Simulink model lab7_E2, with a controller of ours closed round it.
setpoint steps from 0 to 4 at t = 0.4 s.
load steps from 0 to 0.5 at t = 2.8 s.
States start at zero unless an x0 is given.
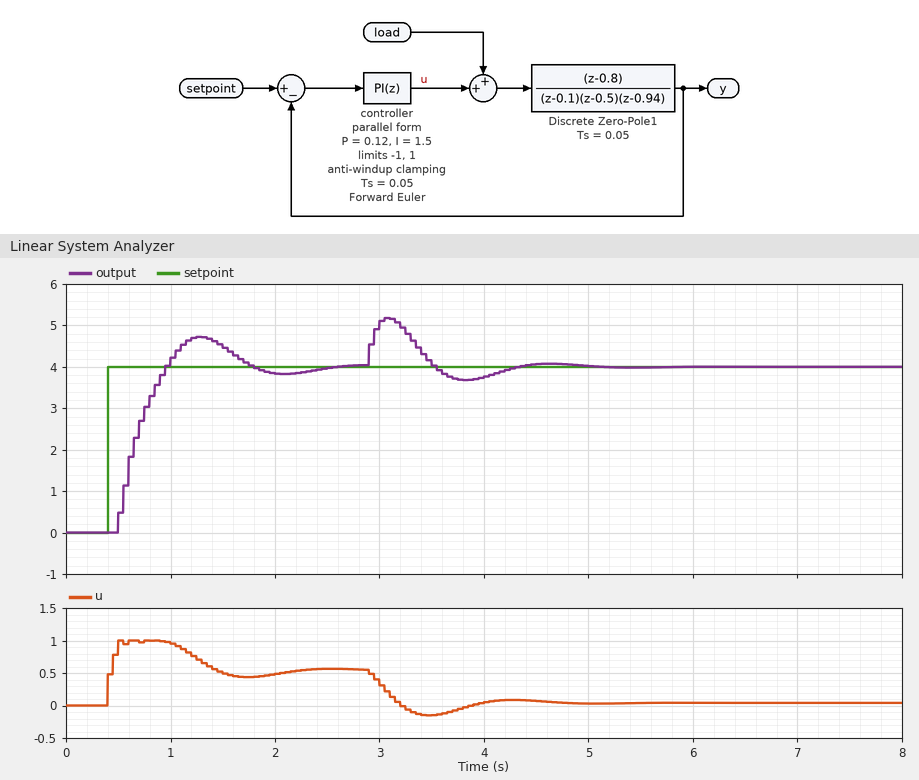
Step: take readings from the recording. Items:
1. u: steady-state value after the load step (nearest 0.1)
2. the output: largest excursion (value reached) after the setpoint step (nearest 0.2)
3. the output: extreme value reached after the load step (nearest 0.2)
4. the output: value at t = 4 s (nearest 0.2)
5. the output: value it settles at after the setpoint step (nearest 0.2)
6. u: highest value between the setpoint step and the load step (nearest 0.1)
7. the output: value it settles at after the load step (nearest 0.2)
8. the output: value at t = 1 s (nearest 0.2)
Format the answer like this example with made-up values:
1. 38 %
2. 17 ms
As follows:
1. 0.0
2. 4.8
3. 5.2
4. 3.8
5. 4.0
6. 1.0
7. 4.0
8. 4.2
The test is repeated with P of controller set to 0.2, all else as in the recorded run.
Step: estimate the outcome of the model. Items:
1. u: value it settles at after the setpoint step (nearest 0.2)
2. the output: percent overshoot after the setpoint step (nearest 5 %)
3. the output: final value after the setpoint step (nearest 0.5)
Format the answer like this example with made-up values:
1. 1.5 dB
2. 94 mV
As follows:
1. 0.6
2. 15 %
3. 4.0
